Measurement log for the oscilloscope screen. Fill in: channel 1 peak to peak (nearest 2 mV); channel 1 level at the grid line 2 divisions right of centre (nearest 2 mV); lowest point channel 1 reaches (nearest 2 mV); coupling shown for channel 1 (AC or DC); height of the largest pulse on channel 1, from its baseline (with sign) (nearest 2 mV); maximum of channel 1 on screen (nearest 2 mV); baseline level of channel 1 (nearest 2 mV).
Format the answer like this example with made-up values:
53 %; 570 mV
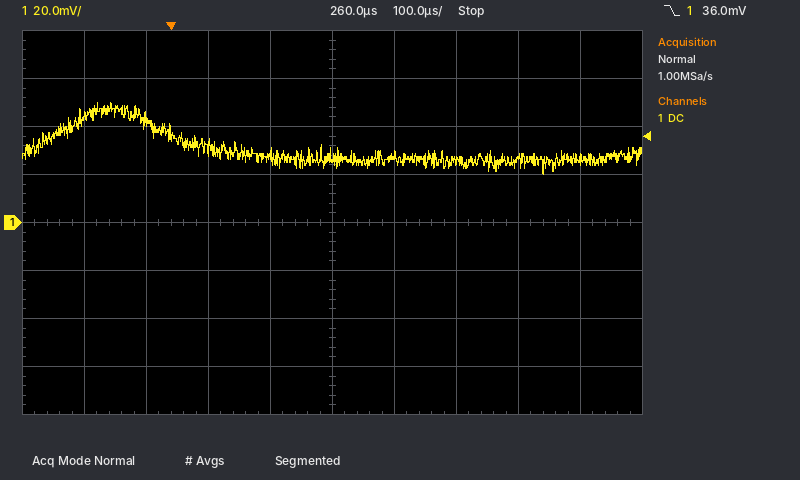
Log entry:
30 mV; 26 mV; 20 mV; DC; +24 mV; 50 mV; 26 mV
